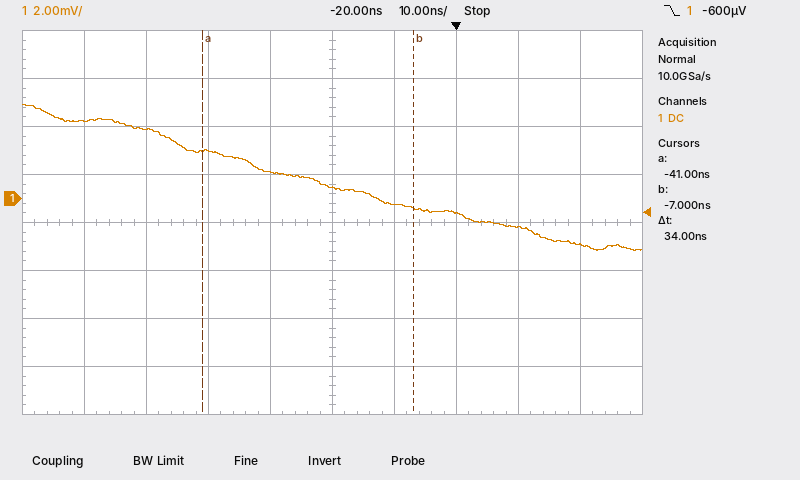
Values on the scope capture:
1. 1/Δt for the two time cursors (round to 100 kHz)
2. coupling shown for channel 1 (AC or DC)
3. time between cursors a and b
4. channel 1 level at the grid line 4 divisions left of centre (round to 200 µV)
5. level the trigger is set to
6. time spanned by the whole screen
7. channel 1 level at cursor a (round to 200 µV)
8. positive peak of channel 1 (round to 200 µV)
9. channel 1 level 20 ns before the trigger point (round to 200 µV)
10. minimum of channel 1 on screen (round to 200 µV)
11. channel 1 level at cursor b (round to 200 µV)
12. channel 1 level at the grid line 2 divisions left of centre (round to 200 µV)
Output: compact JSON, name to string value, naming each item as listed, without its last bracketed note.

{"1/Δt for the two time cursors": "29.4 MHz", "coupling shown for channel 1": "DC", "time between cursors a and b": "34 ns", "channel 1 level at the grid line 4 divisions left of centre": "3.2 mV", "level the trigger is set to": "-600 µV", "time spanned by the whole screen": "100 ns", "channel 1 level at cursor a": "2.0 mV", "positive peak of channel 1": "4.0 mV", "channel 1 level 20 ns before the trigger point": "400 µV", "minimum of channel 1 on screen": "-2.2 mV", "channel 1 level at cursor b": "-400 µV", "channel 1 level at the grid line 2 divisions left of centre": "2.0 mV"}
